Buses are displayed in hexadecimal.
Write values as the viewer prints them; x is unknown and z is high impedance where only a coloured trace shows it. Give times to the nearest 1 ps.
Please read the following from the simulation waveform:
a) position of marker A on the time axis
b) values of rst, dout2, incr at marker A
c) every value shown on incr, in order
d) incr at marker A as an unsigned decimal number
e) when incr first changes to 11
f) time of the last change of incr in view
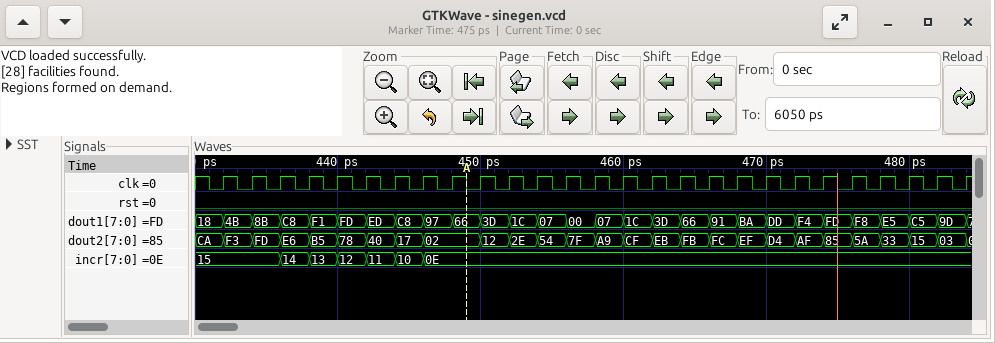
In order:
449 ps
rst=0, dout2=02, incr=0E
15, 14, 13, 12, 11, 10, 0E
14
442 ps
446 ps
